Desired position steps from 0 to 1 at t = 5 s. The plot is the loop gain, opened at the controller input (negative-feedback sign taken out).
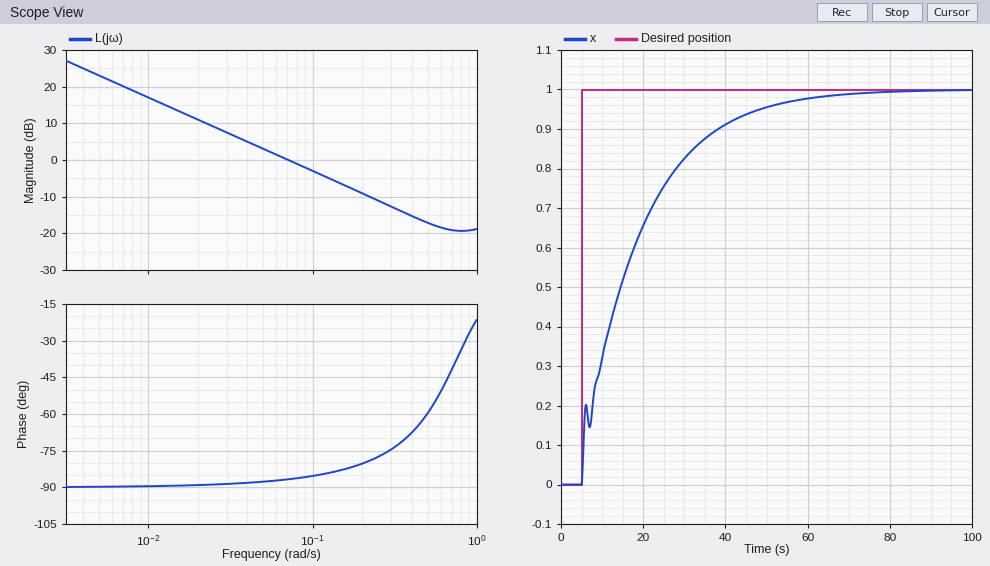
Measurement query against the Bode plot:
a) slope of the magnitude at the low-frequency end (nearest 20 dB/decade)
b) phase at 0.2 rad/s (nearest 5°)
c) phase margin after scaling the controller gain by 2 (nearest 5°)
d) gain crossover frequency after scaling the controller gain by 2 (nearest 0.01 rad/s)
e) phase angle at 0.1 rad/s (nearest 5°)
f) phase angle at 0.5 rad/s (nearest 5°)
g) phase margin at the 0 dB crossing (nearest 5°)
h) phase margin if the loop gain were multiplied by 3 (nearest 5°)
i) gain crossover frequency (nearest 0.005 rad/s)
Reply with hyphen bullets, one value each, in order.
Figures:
- -20 dB/decade
- -80°
- 95°
- 0.14 rad/s
- -85°
- -60°
- 95°
- 100°
- 0.070 rad/s
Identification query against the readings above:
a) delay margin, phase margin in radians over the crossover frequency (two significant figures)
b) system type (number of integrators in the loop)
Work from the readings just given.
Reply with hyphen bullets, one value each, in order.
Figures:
- 24 s
- 1
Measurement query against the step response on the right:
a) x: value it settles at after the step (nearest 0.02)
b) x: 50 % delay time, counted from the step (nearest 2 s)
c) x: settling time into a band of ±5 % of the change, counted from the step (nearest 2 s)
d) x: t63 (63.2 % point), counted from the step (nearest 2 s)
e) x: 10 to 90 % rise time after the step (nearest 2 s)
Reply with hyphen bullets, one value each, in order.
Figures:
- 1.00
- 10 s
- 44 s
- 14 s
- 32 s
